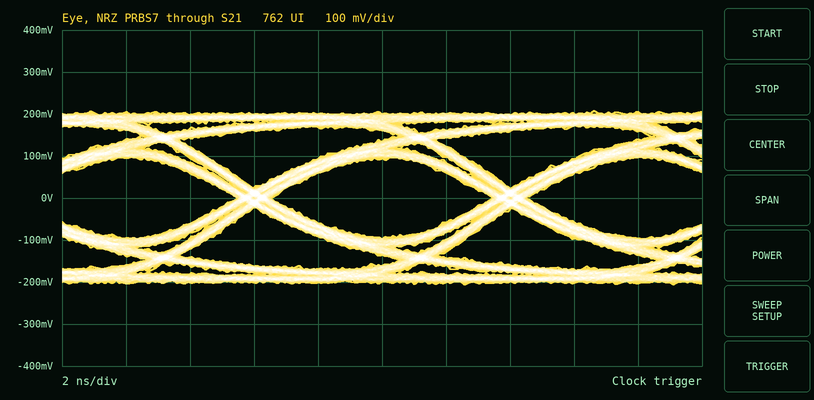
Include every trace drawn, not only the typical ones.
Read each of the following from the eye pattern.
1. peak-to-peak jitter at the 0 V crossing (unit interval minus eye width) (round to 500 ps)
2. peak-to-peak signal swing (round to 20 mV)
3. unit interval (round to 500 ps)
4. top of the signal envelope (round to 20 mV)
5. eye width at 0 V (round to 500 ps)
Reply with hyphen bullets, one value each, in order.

- 1.0 ns
- 420 mV
- 8.0 ns
- 200 mV
- 7.0 ns
